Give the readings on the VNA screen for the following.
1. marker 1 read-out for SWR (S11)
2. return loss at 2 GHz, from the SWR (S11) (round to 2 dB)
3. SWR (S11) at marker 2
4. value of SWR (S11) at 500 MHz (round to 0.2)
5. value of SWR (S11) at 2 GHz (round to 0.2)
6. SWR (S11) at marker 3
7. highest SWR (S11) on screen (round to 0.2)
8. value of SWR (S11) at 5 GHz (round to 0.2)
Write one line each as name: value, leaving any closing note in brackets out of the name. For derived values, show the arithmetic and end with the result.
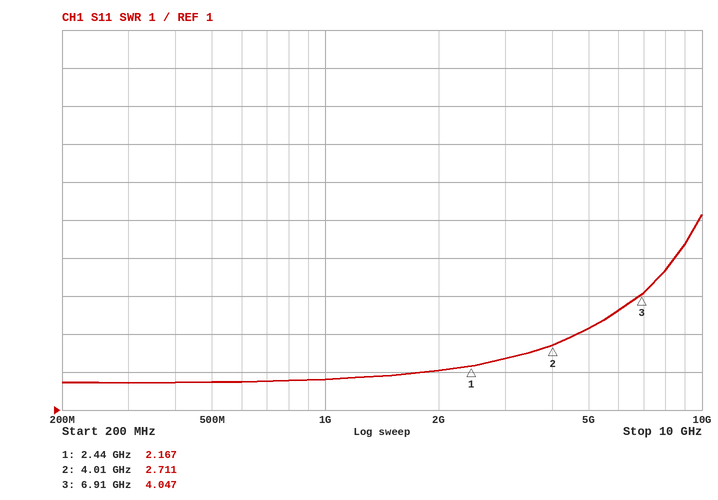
marker 1 read-out for SWR: 2.167
return loss at 2 GHz, from the SWR (S11): −20 log10((2 − 1)/(2 + 1)) ≈ 10 dB
SWR (S11) at marker 2: 2.711
value of SWR (S11) at 500 MHz: 1.8
value of SWR (S11) at 2 GHz: 2.0
SWR (S11) at marker 3: 4.047
highest SWR (S11) on screen: 6.2
value of SWR (S11) at 5 GHz: 3.2
